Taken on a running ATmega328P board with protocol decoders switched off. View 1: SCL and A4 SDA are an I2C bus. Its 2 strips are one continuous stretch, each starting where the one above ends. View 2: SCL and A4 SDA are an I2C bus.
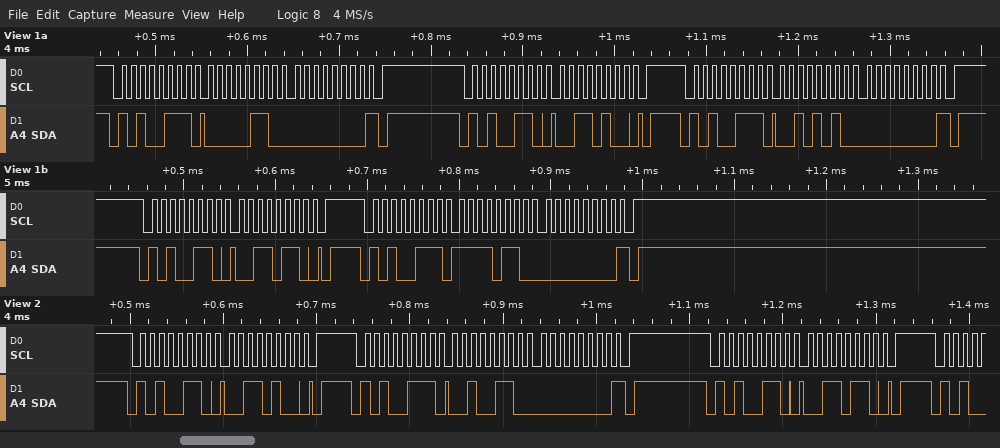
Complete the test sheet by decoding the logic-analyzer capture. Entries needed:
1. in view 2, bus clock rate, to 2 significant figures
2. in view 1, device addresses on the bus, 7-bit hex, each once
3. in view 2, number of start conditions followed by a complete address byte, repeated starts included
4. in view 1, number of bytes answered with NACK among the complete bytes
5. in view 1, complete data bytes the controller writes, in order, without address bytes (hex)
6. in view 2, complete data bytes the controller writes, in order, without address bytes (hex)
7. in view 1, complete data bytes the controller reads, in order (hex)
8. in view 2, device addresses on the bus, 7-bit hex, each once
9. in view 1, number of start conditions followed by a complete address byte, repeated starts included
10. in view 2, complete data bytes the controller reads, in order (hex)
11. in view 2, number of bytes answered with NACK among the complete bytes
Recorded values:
100 kHz
0x53
3
3
34 36
34 36
06 00 2A 00 F6 00
0x53
5
26 00
1
